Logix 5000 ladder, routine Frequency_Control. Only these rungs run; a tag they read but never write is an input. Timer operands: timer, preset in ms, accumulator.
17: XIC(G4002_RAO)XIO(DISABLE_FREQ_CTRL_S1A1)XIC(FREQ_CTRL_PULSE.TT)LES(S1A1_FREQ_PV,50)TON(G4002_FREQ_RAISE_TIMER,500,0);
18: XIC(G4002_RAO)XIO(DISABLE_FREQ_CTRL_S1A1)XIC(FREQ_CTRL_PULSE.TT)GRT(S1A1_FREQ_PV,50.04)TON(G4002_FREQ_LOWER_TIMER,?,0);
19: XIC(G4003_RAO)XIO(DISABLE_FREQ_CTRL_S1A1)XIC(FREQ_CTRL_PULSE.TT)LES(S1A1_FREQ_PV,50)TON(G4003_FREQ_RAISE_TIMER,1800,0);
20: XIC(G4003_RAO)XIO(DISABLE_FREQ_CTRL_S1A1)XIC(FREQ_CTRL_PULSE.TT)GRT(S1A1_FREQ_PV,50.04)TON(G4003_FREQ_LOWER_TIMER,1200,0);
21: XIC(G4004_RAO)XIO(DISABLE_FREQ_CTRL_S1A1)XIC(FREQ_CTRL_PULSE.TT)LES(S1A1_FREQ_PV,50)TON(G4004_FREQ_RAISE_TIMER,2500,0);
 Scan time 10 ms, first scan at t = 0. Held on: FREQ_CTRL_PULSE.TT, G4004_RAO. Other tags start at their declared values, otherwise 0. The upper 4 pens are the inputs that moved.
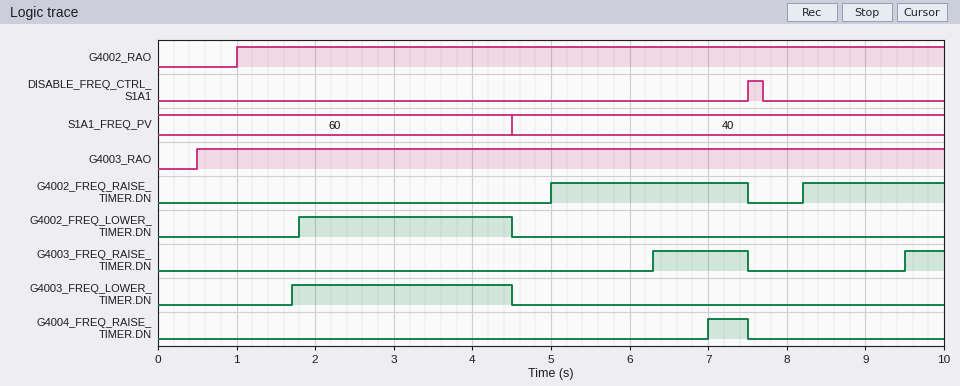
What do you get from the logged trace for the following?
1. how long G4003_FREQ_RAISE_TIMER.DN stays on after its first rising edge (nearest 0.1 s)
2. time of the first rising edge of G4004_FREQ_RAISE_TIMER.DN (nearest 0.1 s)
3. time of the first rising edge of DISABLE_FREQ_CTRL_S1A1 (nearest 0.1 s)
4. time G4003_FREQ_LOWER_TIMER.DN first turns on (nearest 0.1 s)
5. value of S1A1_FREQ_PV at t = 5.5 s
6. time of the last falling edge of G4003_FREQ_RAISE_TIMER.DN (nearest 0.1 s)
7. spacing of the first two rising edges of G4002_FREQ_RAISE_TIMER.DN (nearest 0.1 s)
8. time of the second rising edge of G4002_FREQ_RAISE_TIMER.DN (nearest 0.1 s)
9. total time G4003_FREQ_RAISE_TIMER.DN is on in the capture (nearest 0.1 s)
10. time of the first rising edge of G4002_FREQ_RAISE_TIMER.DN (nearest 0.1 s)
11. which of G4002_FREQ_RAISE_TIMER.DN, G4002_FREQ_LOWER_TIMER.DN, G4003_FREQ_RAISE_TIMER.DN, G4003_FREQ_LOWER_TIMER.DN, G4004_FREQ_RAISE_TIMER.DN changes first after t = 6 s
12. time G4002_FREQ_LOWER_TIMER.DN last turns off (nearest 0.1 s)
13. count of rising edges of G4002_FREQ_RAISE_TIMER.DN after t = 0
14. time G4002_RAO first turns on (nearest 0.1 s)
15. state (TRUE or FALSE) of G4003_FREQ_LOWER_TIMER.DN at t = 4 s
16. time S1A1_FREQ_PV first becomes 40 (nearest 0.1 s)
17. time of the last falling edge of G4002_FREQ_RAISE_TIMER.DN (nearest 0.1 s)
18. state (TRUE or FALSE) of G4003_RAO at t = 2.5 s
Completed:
1.2 s
7.0 s
7.5 s
1.7 s
40
7.5 s
3.2 s
8.2 s
1.7 s
5.0 s
G4003_FREQ_RAISE_TIMER.DN
4.5 s
2
1.0 s
TRUE
4.5 s
7.5 s
TRUE
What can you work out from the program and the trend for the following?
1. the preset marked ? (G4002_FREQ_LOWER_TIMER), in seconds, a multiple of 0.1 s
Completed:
0.8 s
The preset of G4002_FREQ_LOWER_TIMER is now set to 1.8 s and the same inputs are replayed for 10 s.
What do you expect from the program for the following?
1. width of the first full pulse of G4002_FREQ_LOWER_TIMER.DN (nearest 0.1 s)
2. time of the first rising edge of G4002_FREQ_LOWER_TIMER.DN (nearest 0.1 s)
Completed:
1.7 s
2.8 s
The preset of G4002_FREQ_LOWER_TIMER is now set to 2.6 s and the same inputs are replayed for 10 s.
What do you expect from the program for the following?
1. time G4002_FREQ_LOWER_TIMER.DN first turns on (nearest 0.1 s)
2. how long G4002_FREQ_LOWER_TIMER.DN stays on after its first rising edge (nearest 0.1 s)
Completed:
3.6 s
0.9 s
